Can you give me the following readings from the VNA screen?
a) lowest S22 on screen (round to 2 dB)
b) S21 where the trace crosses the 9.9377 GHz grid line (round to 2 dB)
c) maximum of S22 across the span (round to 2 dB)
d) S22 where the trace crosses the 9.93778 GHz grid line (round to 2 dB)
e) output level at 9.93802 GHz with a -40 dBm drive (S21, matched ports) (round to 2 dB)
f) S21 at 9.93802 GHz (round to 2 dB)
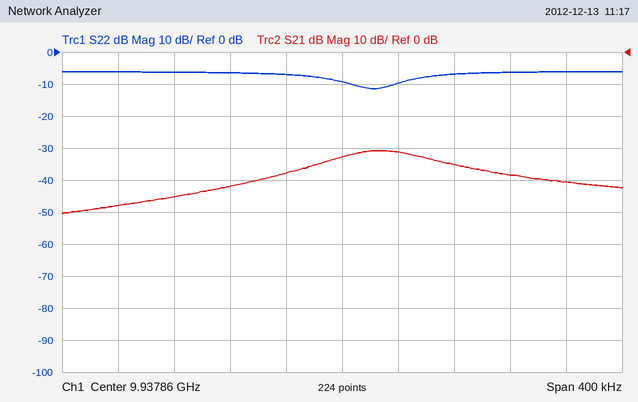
-12 dB
-48 dB
-6 dB
-6 dB
-80 dBm
-40 dB
